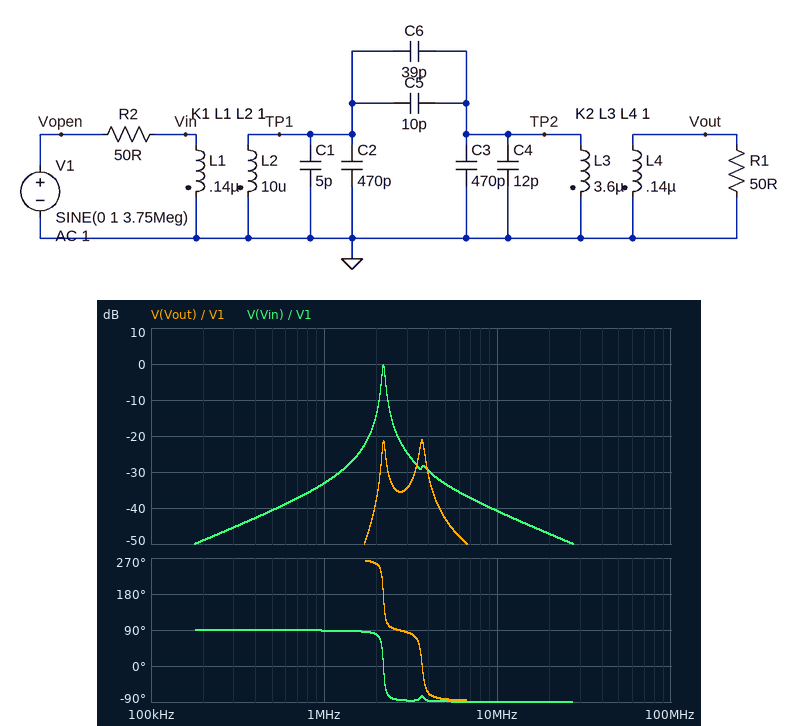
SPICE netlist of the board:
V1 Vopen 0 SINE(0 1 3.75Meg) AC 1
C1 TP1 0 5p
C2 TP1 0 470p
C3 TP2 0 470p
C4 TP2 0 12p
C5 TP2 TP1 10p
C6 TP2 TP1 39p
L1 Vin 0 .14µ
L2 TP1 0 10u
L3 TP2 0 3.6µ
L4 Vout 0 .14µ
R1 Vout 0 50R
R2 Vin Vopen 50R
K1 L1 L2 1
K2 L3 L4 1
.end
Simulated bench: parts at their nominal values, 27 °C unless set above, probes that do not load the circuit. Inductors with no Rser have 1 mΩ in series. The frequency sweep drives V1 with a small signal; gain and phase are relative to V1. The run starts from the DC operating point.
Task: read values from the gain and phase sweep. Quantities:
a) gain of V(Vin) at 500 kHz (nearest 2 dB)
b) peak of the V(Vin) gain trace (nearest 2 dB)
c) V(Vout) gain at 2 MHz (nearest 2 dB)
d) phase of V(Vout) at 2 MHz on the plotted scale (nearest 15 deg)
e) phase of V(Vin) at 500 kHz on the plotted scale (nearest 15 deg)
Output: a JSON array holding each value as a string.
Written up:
["-40 dB", "0 dB", "-38 dB", "255 deg", "90 deg"]
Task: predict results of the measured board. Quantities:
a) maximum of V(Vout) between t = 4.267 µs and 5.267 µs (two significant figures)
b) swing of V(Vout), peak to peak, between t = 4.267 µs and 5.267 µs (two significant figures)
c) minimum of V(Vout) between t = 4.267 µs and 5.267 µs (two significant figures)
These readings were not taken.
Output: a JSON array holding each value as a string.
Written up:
["72 mV", "140 mV", "-72 mV"]
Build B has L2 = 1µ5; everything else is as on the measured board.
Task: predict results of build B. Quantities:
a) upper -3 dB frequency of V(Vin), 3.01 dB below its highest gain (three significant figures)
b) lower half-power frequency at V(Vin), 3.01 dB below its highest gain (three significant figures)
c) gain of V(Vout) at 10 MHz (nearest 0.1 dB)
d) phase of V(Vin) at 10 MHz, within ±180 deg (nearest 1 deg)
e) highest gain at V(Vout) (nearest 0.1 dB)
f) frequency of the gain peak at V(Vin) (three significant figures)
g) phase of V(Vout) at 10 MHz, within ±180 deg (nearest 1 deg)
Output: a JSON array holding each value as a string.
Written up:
["6.01 MHz", "5.44 MHz", "-44.7 dB", "-85 deg", "-20.1 dB", "5.72 MHz", "-84 deg"]
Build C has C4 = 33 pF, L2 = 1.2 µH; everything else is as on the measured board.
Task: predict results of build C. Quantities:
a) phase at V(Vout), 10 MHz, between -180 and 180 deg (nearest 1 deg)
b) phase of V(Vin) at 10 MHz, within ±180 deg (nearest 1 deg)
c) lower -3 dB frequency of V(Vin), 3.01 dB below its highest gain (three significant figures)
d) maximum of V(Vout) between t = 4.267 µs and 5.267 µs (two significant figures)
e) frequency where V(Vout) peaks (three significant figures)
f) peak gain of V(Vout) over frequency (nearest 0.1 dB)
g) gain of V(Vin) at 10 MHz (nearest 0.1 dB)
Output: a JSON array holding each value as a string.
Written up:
["-82 deg", "-83 deg", "6.04 MHz", "44 mV", "6.37 MHz", "-22.6 dB", "-18.4 dB"]
